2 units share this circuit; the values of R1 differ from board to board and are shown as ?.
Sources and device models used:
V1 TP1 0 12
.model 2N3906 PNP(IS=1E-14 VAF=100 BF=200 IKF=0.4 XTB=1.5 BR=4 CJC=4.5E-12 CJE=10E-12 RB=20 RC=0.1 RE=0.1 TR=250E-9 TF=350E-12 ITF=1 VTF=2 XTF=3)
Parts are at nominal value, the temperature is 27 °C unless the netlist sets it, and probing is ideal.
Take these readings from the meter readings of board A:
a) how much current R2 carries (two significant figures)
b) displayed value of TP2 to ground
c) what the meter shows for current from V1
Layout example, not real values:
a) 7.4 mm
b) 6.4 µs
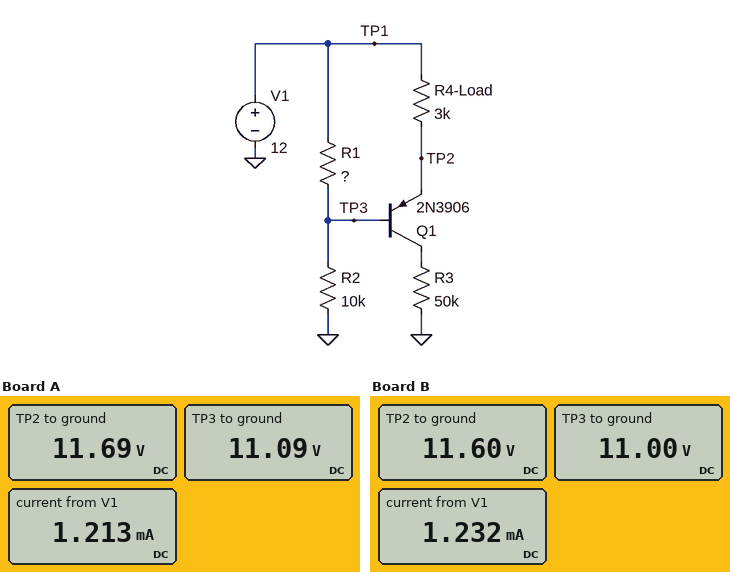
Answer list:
a) 1.1 mA
b) 11.69 V
c) 1.213 mA
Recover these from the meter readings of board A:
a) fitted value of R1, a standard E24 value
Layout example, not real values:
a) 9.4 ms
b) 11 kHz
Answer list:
a) 820 Ω
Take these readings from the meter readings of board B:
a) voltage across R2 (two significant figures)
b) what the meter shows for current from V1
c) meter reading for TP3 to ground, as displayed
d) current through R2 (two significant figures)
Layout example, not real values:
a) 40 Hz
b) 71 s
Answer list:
a) 11 V
b) 1.232 mA
c) 11.00 V
d) 1.1 mA
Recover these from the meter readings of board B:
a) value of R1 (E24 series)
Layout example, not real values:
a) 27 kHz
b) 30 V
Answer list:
a) 910 Ω
